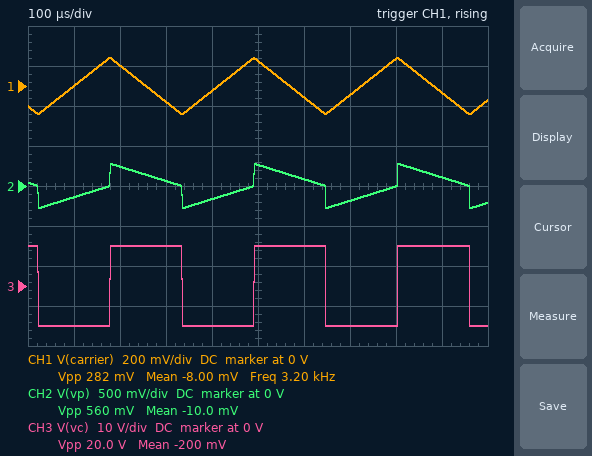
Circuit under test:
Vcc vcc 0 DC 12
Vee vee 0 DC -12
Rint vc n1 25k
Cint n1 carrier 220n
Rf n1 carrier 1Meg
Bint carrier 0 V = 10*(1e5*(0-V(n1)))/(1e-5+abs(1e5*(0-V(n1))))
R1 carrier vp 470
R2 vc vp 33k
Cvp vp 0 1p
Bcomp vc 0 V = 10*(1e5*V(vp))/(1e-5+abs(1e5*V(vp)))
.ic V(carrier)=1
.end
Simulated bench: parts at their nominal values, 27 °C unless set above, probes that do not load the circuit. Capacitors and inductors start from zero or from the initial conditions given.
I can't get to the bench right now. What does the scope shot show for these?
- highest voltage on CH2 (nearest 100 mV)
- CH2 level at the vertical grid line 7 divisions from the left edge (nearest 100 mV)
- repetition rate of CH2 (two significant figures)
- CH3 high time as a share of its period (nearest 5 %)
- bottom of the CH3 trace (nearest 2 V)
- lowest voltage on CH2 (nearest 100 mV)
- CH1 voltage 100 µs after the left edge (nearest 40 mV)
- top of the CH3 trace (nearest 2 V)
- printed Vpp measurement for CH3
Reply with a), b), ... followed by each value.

a) 300 mV
b) -200 mV
c) 3.2 kHz
d) 50 %
e) -10 V
f) -300 mV
g) 0 V
h) 10 V
i) 20.0 V
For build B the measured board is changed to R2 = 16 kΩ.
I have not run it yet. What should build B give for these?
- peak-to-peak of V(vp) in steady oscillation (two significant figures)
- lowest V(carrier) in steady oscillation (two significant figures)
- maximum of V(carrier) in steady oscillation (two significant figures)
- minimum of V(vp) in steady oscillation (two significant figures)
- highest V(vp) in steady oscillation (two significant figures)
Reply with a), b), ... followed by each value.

a) 1.1 V
b) -290 mV
c) 290 mV
d) -570 mV
e) 570 mV
